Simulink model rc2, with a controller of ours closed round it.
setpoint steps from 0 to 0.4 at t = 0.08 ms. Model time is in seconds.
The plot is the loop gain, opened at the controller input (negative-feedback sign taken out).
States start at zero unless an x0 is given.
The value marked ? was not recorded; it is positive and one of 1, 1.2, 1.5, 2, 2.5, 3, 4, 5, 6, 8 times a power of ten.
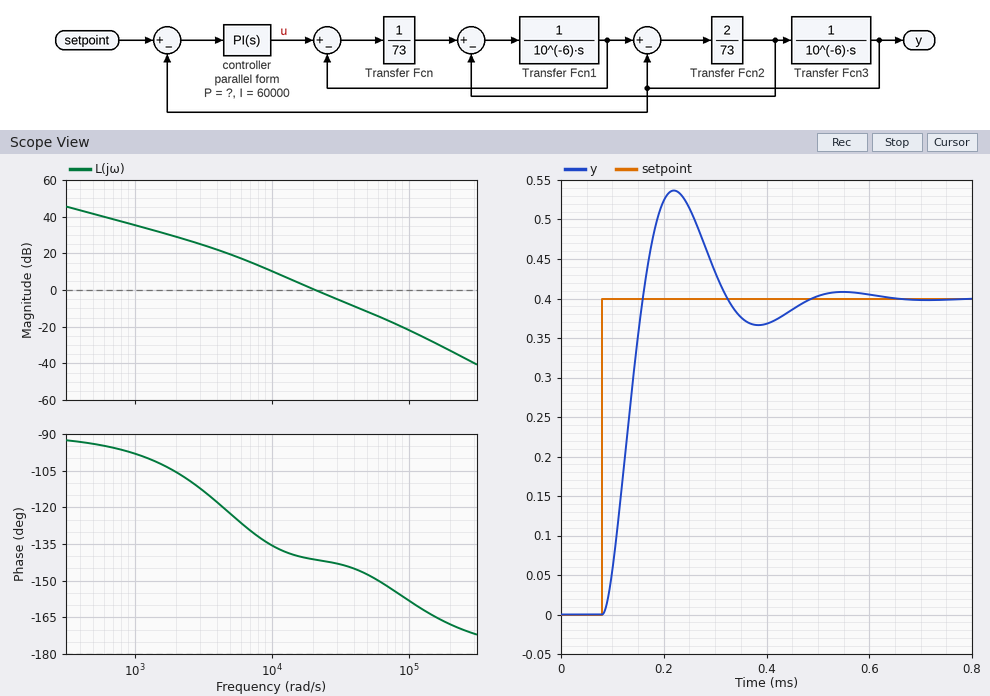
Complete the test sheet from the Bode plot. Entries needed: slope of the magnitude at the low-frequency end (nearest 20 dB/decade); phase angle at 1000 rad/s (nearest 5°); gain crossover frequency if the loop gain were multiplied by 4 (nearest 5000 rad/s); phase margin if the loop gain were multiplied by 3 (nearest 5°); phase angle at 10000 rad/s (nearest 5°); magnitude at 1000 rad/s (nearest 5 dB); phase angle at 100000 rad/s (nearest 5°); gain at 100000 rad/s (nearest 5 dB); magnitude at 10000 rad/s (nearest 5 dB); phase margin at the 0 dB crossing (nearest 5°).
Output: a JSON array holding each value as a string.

["-20 dB/decade", "-100°", "50000 rad/s", "35°", "-135°", "35 dB", "-160°", "-20 dB", "10 dB", "40°"]
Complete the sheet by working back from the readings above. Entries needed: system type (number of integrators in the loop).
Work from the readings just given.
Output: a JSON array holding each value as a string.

["1"]
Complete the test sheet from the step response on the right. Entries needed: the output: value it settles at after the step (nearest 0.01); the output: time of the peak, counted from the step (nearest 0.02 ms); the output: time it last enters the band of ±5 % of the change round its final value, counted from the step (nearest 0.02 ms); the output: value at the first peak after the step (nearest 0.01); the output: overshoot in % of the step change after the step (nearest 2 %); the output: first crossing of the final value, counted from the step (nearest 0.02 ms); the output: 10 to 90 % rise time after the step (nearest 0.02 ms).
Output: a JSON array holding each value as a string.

["0.40", "0.14 ms", "0.36 ms", "0.54", "34 %", "0.08 ms", "0.06 ms"]
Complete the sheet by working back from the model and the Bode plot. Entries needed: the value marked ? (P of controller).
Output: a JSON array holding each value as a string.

["2.5"]
